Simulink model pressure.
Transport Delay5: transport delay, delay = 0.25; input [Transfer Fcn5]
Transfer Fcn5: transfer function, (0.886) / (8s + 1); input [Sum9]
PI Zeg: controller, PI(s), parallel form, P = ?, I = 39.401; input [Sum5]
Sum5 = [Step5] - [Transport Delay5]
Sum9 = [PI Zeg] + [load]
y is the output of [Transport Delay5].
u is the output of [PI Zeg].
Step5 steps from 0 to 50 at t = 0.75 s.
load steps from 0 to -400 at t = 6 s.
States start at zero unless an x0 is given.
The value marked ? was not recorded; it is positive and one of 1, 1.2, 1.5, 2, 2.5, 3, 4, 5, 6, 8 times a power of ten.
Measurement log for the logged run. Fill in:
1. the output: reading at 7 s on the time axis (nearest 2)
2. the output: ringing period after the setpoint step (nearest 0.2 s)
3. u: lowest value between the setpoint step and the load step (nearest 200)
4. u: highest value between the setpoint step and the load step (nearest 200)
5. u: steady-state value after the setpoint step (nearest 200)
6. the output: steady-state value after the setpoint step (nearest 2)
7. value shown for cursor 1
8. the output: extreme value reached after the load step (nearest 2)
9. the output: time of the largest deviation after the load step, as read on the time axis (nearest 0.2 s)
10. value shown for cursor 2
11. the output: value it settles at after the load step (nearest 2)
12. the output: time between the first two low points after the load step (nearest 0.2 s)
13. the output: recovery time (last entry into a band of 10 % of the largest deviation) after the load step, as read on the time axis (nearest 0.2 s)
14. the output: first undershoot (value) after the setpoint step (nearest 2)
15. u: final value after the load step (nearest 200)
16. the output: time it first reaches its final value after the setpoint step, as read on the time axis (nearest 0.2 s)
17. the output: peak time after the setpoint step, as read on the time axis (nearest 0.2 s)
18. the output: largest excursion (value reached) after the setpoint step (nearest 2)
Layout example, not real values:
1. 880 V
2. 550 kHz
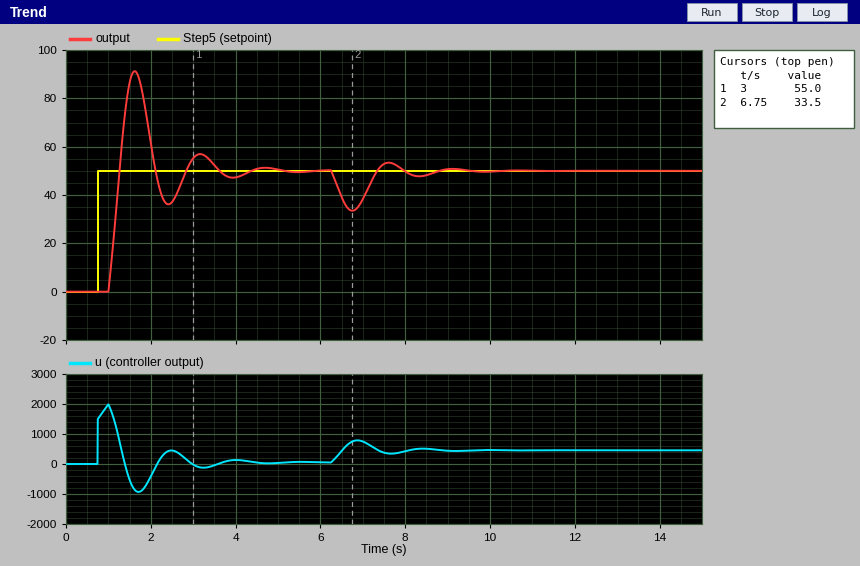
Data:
1. 38
2. 1.6 s
3. -1000
4. 2000
5. 0
6. 50
7. 55.0
8. 34
9. 6.8 s
10. 33.5
11. 50
12. 1.6 s
13. 8.6 s
14. 36
15. 400
16. 1.2 s
17. 1.6 s
18. 92
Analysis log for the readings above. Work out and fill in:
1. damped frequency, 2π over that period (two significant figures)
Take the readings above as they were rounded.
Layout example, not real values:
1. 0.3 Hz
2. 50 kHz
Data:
1. 3.9 rad/s
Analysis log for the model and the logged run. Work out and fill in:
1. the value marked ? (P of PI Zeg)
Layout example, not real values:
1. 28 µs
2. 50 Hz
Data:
1. 30
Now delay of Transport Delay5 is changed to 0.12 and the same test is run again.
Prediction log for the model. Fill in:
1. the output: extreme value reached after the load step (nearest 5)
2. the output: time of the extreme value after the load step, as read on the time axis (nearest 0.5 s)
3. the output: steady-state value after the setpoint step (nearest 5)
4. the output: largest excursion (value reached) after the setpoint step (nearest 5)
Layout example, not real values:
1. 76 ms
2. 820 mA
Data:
1. 40
2. 6.5 s
3. 50
4. 65
